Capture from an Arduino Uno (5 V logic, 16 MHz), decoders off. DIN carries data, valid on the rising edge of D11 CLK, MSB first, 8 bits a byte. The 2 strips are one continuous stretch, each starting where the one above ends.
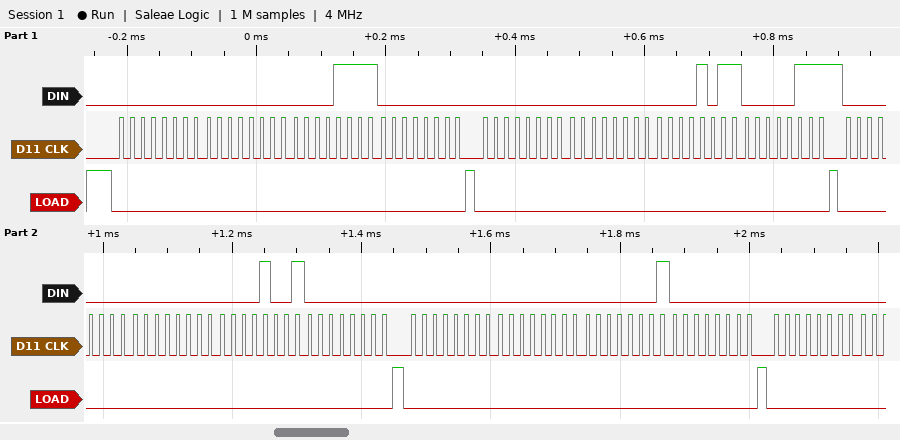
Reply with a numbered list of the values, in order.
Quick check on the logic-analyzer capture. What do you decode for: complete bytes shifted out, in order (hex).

1. 00 00 0F 00 00 00 0B 07 00 00 09 00 00 00 01 00 00
